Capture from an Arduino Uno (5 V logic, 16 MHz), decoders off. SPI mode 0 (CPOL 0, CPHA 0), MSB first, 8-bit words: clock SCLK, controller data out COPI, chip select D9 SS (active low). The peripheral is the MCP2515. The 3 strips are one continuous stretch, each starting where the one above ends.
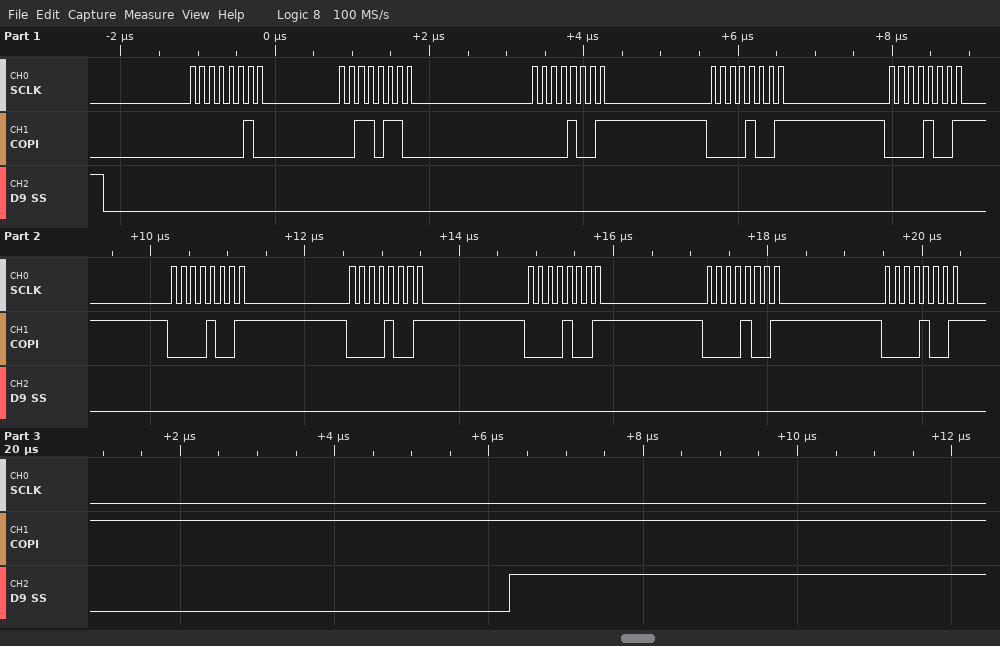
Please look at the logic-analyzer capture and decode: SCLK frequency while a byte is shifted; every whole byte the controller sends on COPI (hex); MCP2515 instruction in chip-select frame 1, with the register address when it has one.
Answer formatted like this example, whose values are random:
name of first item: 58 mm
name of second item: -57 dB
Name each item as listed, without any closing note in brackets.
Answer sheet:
SCLK frequency while a byte is shifted: 8 MHz
every whole byte the controller sends on COPI: 0x02 0x36 0x09 0x09 0x09 0x09 0x09 0x09 0x09 0x09
MCP2515 instruction in chip-select frame 1, with the register address when it has one: WRITE 0x36
